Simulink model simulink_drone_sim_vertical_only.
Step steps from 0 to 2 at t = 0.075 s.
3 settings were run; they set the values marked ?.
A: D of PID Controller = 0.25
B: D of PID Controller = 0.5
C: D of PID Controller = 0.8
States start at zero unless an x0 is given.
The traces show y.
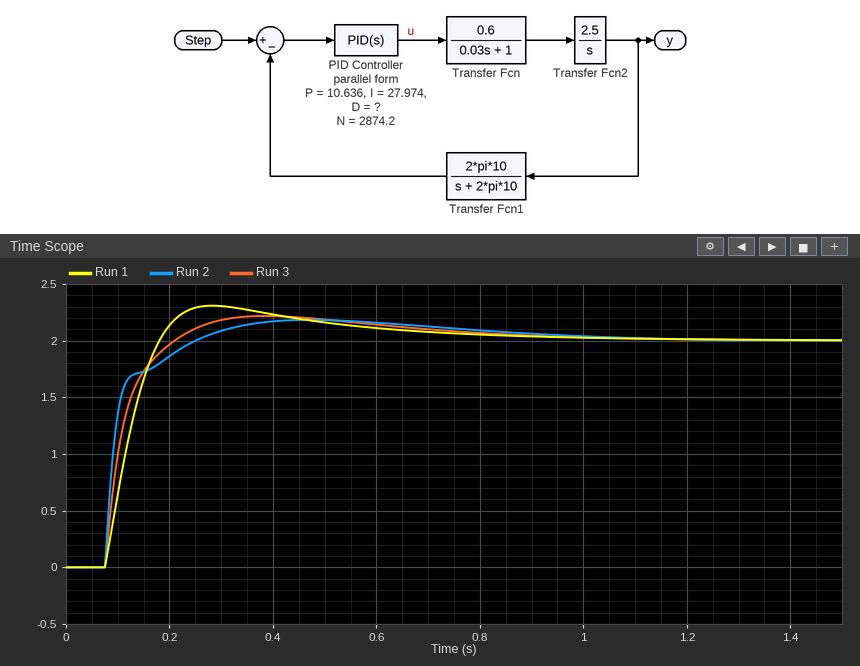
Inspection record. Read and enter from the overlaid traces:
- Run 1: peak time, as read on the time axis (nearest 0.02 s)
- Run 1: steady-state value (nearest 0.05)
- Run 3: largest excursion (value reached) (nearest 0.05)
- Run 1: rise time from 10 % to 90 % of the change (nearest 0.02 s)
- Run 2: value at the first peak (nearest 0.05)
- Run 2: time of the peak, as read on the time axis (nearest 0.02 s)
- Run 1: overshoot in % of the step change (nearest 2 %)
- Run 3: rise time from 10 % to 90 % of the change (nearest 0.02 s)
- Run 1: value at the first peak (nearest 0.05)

0.28 s
2.00
2.20
0.08 s
2.20
0.48 s
16 %
0.08 s
2.30
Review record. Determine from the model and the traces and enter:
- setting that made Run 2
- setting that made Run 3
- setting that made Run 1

C
B
A
